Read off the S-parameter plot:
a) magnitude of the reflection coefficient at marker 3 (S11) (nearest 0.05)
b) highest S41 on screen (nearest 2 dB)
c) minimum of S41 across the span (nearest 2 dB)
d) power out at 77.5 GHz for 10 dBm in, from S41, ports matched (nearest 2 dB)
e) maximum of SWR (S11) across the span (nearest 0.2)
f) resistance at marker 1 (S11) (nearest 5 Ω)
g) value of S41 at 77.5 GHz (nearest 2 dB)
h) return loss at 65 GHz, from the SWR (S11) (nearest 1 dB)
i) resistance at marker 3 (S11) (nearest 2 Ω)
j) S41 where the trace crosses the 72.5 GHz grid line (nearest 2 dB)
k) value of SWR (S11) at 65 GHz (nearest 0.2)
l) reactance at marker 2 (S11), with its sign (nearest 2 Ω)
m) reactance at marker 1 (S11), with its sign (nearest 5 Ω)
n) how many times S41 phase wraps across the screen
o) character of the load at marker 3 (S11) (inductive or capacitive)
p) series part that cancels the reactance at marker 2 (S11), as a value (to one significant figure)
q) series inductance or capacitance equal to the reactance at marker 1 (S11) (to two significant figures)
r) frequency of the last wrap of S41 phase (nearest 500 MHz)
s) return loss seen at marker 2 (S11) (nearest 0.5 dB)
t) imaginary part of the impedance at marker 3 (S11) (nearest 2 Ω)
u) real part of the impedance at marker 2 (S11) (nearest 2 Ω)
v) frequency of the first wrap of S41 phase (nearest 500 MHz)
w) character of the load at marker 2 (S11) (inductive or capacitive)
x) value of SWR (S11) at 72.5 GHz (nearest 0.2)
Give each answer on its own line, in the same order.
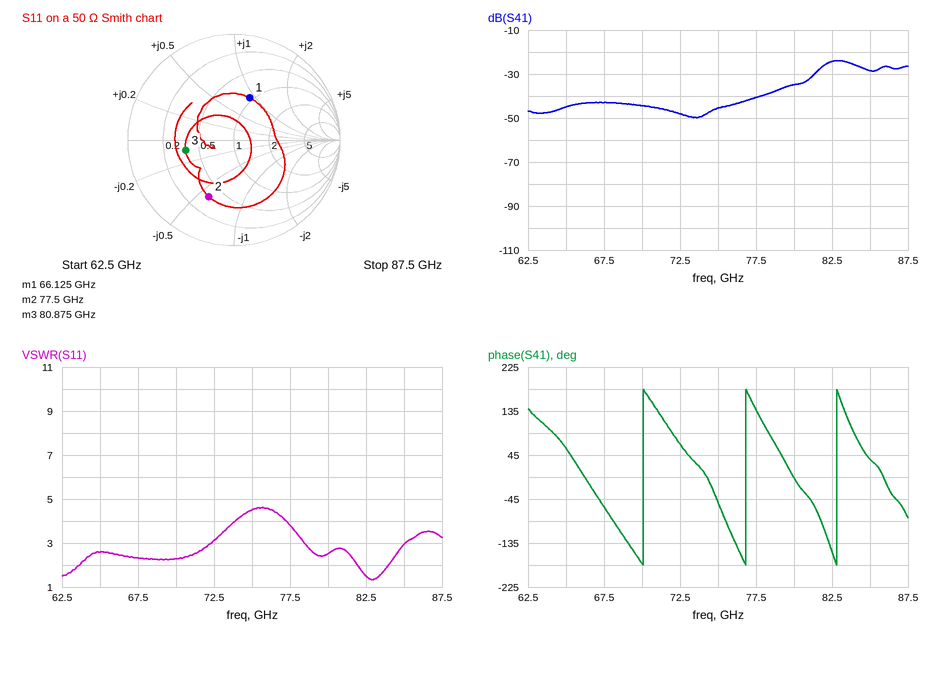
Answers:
0.45
-24 dB
-50 dB
-30 dBm
4.6
45 Ω
-40 dB
7 dB
18 Ω
-48 dB
2.6
-30 Ω
+45 Ω
3
capacitive
60 pH
110 pH
83.0 GHz
4.5 dB
-4 Ω
18 Ω
70.0 GHz
capacitive
3.2
